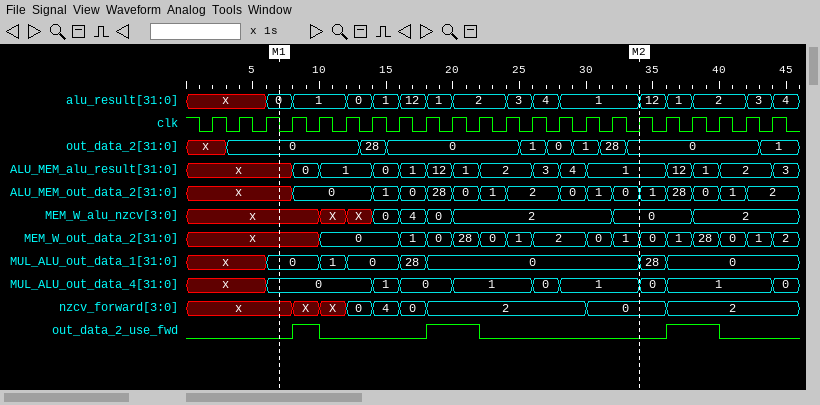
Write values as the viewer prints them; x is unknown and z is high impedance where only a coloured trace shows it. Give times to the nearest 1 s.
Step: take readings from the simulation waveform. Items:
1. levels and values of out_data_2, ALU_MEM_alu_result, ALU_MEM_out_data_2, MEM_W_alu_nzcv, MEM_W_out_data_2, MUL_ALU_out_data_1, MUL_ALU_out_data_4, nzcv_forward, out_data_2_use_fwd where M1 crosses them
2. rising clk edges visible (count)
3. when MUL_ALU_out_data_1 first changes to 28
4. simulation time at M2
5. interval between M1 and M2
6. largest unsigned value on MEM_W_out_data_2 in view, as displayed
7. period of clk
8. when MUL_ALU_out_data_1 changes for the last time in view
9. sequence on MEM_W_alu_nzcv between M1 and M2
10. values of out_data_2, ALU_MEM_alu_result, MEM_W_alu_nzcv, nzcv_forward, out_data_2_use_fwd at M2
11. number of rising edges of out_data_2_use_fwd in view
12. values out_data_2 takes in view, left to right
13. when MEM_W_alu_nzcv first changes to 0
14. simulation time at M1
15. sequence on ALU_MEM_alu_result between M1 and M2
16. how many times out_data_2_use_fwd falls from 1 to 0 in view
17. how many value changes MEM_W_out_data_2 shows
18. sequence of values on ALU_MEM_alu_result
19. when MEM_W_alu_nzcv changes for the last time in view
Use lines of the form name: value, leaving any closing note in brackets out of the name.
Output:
levels and values of out_data_2, ALU_MEM_alu_result, ALU_MEM_out_data_2, MEM_W_alu_nzcv, MEM_W_out_data_2, MUL_ALU_out_data_1, MUL_ALU_out_data_4, nzcv_forward, out_data_2_use_fwd where M1 crosses them: out_data_2=0, ALU_MEM_alu_result=x, ALU_MEM_out_data_2=x, MEM_W_alu_nzcv=x, MEM_W_out_data_2=x, MUL_ALU_out_data_1=0, MUL_ALU_out_data_4=0, nzcv_forward=x, out_data_2_use_fwd=0
rising clk edges visible: 22
when MUL_ALU_out_data_1 first changes to 28: 16 s
simulation time at M2: 34 s
interval between M1 and M2: 27 s
largest unsigned value on MEM_W_out_data_2 in view, as displayed: 28
period of clk: 2 s
when MUL_ALU_out_data_1 changes for the last time in view: 36 s
sequence on MEM_W_alu_nzcv between M1 and M2: x, X, X, 0, 4, 0, 2, 0
values of out_data_2, ALU_MEM_alu_result, MEM_W_alu_nzcv, nzcv_forward, out_data_2_use_fwd at M2: out_data_2=0, ALU_MEM_alu_result=1, MEM_W_alu_nzcv=0, nzcv_forward=0, out_data_2_use_fwd=0
number of rising edges of out_data_2_use_fwd in view: 3
values out_data_2 takes in view, left to right: x, 0, 28, 0, 1, 0, 1, 28, 0, 1
when MEM_W_alu_nzcv first changes to 0: 14 s
simulation time at M1: 7 s
sequence on ALU_MEM_alu_result between M1 and M2: x, 0, 1, 0, 1, 12, 1, 2, 3, 4, 1
how many times out_data_2_use_fwd falls from 1 to 0 in view: 3
how many value changes MEM_W_out_data_2 shows: 15
sequence of values on ALU_MEM_alu_result: x, 0, 1, 0, 1, 12, 1, 2, 3, 4, 1, 12, 1, 2, 3
when MEM_W_alu_nzcv changes for the last time in view: 38 s
